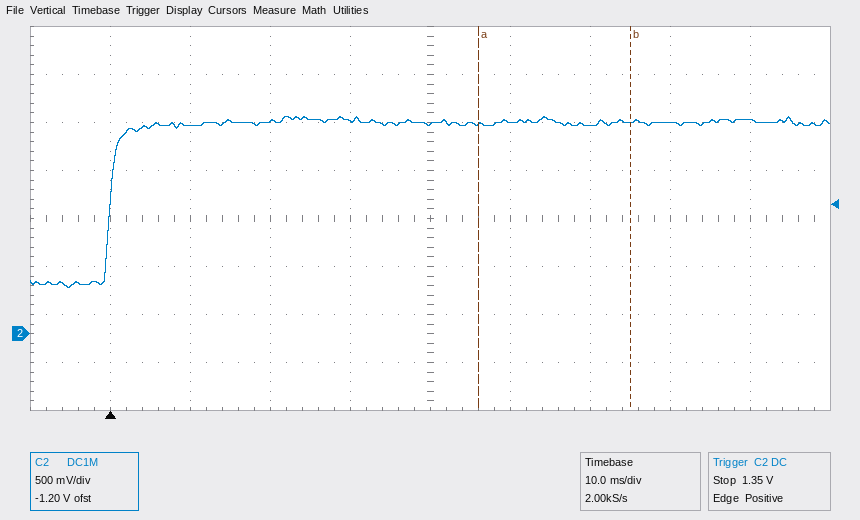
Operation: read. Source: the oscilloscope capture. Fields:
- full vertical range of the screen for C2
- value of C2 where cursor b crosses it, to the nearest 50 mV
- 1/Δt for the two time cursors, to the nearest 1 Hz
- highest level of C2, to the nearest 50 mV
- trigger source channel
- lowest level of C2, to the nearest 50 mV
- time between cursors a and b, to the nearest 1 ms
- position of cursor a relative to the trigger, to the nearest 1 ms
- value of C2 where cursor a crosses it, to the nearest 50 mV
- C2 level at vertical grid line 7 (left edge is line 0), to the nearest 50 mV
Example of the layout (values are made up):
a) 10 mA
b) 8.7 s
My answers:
a) 4 V
b) 2.20 V
c) 53 Hz
d) 2.25 V
e) C2
f) 500 mV
g) 19 ms
h) +46 ms
i) 2.20 V
j) 2.15 V
